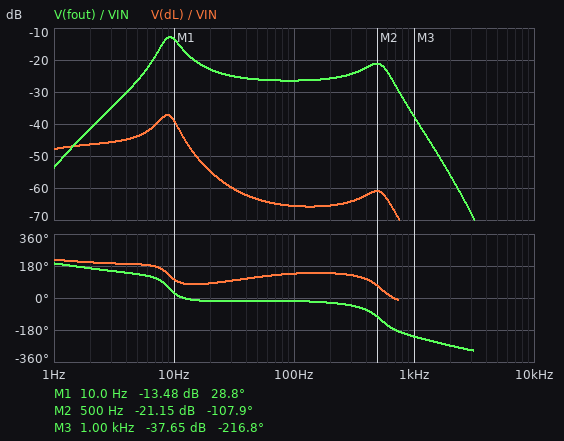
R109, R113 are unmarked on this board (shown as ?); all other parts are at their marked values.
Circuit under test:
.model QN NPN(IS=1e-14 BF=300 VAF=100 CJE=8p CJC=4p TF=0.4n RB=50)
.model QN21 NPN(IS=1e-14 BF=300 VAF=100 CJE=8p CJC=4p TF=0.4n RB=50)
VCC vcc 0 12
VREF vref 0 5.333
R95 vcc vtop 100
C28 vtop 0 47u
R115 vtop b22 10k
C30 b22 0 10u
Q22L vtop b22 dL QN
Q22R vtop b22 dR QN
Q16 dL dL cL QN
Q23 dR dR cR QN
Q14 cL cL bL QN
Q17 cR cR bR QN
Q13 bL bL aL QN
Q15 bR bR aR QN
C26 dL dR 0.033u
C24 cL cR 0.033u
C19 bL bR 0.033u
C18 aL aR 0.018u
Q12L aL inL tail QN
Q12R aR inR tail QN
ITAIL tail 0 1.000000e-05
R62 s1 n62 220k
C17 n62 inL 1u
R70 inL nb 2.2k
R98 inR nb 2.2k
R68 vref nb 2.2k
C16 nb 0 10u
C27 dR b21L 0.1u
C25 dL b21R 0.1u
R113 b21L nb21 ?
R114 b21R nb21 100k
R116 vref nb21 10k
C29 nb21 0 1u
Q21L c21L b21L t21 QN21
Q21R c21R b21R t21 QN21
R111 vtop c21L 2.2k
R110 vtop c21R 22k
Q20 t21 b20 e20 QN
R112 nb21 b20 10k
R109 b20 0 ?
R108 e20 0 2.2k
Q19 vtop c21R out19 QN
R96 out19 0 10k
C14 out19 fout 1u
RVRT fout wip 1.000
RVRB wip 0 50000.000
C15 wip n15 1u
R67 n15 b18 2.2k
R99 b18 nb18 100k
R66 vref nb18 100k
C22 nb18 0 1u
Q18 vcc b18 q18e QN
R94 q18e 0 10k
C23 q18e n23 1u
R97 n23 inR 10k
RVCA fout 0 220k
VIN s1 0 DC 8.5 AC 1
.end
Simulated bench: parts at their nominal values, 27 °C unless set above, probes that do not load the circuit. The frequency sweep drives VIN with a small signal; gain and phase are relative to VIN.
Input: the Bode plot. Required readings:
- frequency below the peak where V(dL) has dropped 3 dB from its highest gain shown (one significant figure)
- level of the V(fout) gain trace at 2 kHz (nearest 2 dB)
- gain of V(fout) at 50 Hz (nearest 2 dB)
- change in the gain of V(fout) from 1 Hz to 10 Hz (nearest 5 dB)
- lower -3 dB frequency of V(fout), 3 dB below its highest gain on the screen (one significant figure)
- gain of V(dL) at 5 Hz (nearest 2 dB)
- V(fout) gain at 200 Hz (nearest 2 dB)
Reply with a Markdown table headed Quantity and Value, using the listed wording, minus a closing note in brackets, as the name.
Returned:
| Quantity | Value |
|---|---|
| frequency below the peak where V(dL) has dropped 3 dB from its highest gain shown | 7 Hz |
| level of the V(fout) gain trace at 2 kHz | -56 dB |
| gain of V(fout) at 50 Hz | -26 dB |
| change in the gain of V(fout) from 1 Hz to 10 Hz | 40 dB |
| lower -3 dB frequency of V(fout), 3 dB below its highest gain on the screen | 8 Hz |
| gain of V(dL) at 5 Hz | -44 dB |
| V(fout) gain at 200 Hz | -26 dB |
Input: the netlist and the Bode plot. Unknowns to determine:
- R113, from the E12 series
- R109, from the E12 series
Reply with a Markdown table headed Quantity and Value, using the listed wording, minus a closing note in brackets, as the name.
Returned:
| Quantity | Value |
|---|---|
| R113, from the E12 series | 68 kΩ |
| R109, from the E12 series | 5.6 kΩ |
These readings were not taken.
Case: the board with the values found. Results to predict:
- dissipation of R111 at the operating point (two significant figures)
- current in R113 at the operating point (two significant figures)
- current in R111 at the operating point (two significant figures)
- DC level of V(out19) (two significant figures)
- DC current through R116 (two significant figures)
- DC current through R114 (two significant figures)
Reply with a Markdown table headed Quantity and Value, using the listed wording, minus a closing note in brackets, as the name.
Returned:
| Quantity | Value |
|---|---|
| dissipation of R111 at the operating point | 41 µW |
| current in R113 at the operating point | 420 nA |
| current in R111 at the operating point | 140 µA |
| DC level of V(out19) | 8.8 V |
| DC current through R116 | 210 µA |
| DC current through R114 | 340 nA |
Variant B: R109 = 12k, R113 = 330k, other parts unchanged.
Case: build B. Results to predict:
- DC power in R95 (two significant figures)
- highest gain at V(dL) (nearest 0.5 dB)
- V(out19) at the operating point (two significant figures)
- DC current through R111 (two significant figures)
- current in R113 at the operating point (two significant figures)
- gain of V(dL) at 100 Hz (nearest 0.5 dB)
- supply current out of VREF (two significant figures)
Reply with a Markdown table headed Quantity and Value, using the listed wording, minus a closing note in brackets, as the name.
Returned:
| Quantity | Value |
|---|---|
| DC power in R95 | 72 µW |
| highest gain at V(dL) | -45.5 dB |
| V(out19) at the operating point | 2.4 V |
| DC current through R111 | 200 µA |
| current in R113 at the operating point | 610 nA |
| gain of V(dL) at 100 Hz | -54.0 dB |
| supply current out of VREF | 170 µA |
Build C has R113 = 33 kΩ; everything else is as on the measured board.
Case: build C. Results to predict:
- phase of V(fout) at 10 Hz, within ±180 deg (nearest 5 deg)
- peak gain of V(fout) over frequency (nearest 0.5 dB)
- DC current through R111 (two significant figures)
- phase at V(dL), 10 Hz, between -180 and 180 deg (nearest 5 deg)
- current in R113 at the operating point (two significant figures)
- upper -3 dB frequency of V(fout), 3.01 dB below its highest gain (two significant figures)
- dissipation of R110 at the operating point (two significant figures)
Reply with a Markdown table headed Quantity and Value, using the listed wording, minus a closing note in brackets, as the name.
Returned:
| Quantity | Value |
|---|---|
| phase of V(fout) at 10 Hz, within ±180 deg | 45 deg |
| peak gain of V(fout) over frequency | -15.0 dB |
| DC current through R111 | 150 µA |
| phase at V(dL), 10 Hz, between -180 and 180 deg | 120 deg |
| current in R113 at the operating point | 470 nA |
| upper -3 dB frequency of V(fout), 3.01 dB below its highest gain | 13 Hz |
| dissipation of R110 at the operating point | 200 µW |
